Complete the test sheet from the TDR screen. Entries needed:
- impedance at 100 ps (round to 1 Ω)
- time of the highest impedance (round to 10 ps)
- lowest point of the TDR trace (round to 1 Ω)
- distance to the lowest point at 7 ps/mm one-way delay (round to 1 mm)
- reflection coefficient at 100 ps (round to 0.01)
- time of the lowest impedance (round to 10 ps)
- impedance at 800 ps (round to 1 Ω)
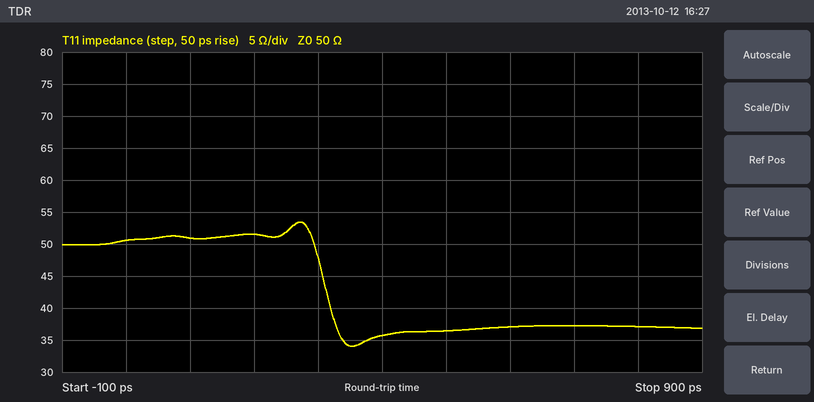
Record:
51 Ω
270 ps
34 Ω
25 mm
+0.01
350 ps
37 Ω
